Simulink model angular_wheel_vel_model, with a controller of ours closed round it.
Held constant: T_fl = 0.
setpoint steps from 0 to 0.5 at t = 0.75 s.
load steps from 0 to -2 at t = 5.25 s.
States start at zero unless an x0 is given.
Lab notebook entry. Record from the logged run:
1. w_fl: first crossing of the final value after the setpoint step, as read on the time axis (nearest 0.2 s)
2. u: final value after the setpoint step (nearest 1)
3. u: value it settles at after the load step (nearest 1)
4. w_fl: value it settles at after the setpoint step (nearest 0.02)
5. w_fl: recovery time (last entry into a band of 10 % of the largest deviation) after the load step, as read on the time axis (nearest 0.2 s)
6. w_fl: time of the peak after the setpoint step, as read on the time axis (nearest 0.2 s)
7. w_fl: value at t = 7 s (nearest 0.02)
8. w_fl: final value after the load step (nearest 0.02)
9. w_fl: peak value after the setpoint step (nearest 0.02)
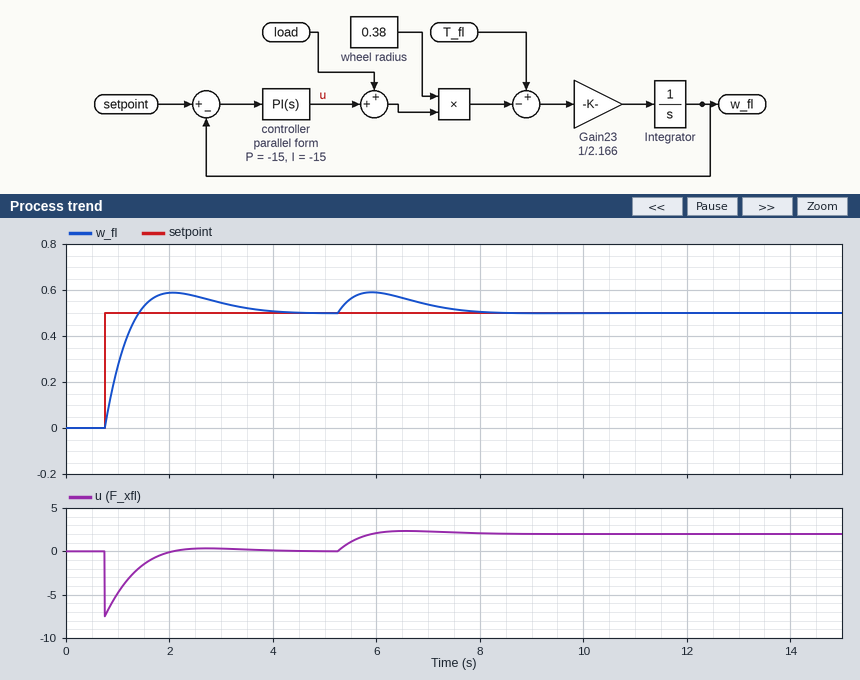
1.4 s
0
2
0.50
7.8 s
2.0 s
0.54
0.50
0.58
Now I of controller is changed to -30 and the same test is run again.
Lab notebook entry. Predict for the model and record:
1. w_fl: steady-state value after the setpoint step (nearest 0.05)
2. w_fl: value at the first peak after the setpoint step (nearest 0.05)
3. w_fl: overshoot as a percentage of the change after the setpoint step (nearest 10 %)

0.50
0.65
30 %
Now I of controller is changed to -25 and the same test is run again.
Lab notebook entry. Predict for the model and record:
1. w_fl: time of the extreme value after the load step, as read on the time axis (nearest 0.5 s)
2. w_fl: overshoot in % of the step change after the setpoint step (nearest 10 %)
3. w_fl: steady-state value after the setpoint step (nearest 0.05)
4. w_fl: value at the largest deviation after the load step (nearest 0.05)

6.0 s
20 %
0.50
0.60
